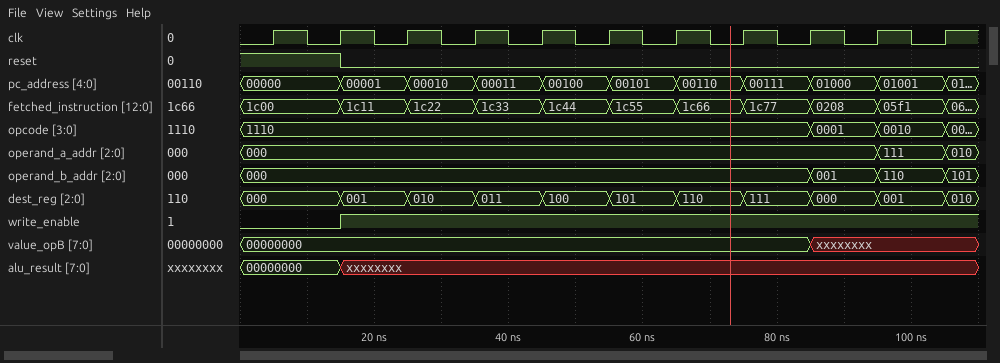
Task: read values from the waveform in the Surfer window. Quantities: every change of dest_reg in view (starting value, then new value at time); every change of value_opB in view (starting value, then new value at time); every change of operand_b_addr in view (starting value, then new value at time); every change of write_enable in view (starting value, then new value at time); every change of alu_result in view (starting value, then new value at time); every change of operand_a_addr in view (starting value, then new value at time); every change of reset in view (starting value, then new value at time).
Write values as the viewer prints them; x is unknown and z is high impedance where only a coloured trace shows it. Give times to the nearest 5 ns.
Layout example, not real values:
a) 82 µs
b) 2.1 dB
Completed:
a) 000, 001 at 15 ns, 010 at 25 ns, 011 at 35 ns, 100 at 45 ns, 101 at 55 ns, 110 at 65 ns, 111 at 75 ns, 000 at 85 ns, 001 at 95 ns, 010 at 105 ns
b) 00000000, xxxxxxxx at 85 ns
c) 000, 001 at 85 ns, 110 at 95 ns, 101 at 105 ns
d) 0, 1 at 15 ns
e) 00000000, xxxxxxxx at 15 ns
f) 000, 111 at 95 ns, 010 at 105 ns
g) 1, 0 at 15 ns
